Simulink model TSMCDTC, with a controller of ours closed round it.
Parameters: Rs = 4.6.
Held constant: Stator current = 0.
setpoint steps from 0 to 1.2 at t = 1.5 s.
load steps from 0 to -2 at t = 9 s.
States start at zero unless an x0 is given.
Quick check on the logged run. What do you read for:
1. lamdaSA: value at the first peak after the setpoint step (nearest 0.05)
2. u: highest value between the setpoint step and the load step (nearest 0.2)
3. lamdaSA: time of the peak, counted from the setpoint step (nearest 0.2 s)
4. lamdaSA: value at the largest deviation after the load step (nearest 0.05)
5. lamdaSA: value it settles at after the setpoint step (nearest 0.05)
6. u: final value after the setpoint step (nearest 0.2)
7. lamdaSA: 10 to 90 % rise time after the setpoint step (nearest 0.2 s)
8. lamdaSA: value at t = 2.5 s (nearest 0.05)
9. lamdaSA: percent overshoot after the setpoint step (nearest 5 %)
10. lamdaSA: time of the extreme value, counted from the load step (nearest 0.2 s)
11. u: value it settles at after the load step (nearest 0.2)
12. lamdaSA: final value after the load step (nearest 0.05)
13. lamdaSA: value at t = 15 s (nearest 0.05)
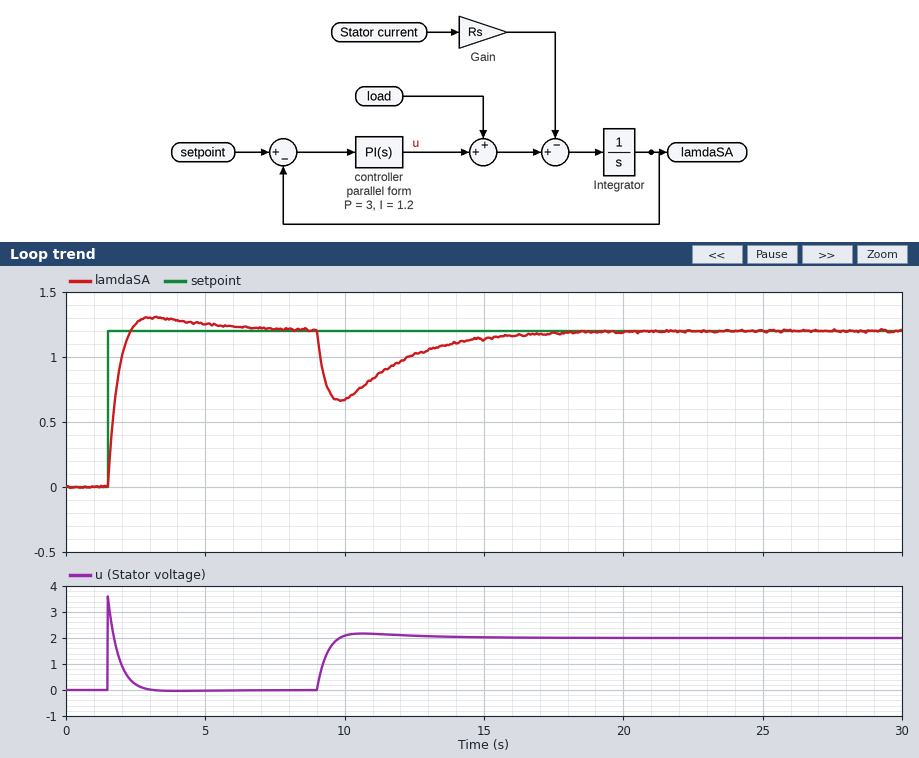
1.30
3.6
1.6 s
0.65
1.20
0.0
0.6 s
1.25
10 %
0.8 s
2.0
1.20
1.15
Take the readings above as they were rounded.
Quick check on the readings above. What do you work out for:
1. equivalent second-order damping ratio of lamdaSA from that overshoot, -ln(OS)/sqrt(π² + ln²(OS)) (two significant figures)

0.59
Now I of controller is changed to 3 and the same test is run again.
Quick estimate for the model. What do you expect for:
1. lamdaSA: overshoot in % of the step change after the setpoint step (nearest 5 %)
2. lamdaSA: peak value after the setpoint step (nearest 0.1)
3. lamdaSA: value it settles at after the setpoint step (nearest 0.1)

15 %
1.4
1.2
